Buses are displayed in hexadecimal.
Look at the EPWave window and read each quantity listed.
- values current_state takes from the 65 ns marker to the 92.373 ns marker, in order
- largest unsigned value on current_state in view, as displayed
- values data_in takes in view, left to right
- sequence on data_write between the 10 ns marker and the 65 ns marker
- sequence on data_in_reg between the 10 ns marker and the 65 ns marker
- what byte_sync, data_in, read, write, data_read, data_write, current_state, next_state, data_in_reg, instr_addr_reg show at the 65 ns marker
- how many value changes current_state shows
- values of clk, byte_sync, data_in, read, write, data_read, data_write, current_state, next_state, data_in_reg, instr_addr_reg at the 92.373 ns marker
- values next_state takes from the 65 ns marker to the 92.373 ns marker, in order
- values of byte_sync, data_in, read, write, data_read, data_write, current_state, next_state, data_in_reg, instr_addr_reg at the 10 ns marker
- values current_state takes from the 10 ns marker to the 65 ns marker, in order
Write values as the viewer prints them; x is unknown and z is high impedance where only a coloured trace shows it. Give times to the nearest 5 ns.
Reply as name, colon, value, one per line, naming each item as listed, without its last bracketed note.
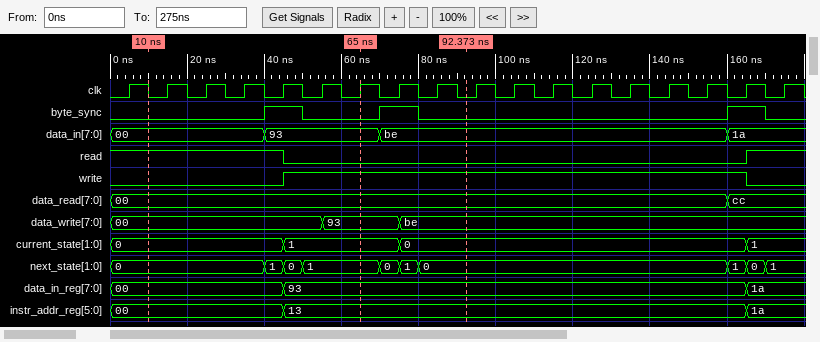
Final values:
values current_state takes from the 65 ns marker to the 92.373 ns marker, in order: 1, 0
largest unsigned value on current_state in view, as displayed: 1
values data_in takes in view, left to right: 00, 93, be, 1a
sequence on data_write between the 10 ns marker and the 65 ns marker: 00, 93
sequence on data_in_reg between the 10 ns marker and the 65 ns marker: 00, 93
what byte_sync, data_in, read, write, data_read, data_write, current_state, next_state, data_in_reg, instr_addr_reg show at the 65 ns marker: byte_sync=0, data_in=93, read=0, write=1, data_read=00, data_write=93, current_state=1, next_state=1, data_in_reg=93, instr_addr_reg=13
how many value changes current_state shows: 3
values of clk, byte_sync, data_in, read, write, data_read, data_write, current_state, next_state, data_in_reg, instr_addr_reg at the 92.373 ns marker: clk=0, byte_sync=0, data_in=be, read=0, write=1, data_read=00, data_write=be, current_state=0, next_state=0, data_in_reg=93, instr_addr_reg=13
values next_state takes from the 65 ns marker to the 92.373 ns marker, in order: 1, 0, 1, 0
values of byte_sync, data_in, read, write, data_read, data_write, current_state, next_state, data_in_reg, instr_addr_reg at the 10 ns marker: byte_sync=0, data_in=00, read=1, write=0, data_read=00, data_write=00, current_state=0, next_state=0, data_in_reg=00, instr_addr_reg=00
values current_state takes from the 10 ns marker to the 65 ns marker, in order: 0, 1
